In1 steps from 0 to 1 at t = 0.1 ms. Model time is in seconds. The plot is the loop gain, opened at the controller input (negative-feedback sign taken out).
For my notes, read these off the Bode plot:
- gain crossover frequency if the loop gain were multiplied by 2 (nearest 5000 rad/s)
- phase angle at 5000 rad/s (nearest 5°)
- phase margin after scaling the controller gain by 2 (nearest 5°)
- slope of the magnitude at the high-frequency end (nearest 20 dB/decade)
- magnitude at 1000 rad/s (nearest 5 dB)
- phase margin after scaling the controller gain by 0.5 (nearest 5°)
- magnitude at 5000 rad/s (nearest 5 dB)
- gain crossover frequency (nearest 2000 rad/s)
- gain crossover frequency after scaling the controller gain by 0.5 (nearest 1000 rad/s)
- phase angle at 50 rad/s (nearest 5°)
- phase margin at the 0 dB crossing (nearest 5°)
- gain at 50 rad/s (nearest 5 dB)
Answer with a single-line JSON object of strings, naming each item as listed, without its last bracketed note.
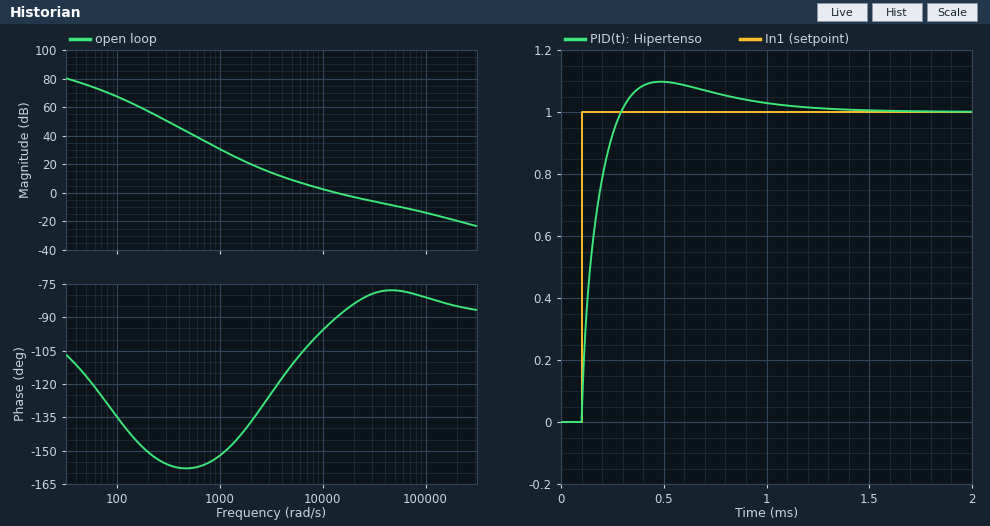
{"gain crossover frequency if the loop gain were multiplied by 2": "30000 rad/s", "phase angle at 5000 rad/s": "-110°", "phase margin after scaling the controller gain by 2": "100°", "slope of the magnitude at the high-frequency end": "-20 dB/decade", "magnitude at 1000 rad/s": "30 dB", "phase margin after scaling the controller gain by 0.5": "75°", "magnitude at 5000 rad/s": "10 dB", "gain crossover frequency": "14000 rad/s", "gain crossover frequency after scaling the controller gain by 0.5": "7000 rad/s", "phase angle at 50 rad/s": "-115°", "phase margin at the 0 dB crossing": "90°", "gain at 50 rad/s": "75 dB"}
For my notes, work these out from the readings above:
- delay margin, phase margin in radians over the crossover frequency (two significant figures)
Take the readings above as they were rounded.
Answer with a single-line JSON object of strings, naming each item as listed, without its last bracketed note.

{"delay margin, phase margin in radians over the crossover frequency": "0.00011 s"}
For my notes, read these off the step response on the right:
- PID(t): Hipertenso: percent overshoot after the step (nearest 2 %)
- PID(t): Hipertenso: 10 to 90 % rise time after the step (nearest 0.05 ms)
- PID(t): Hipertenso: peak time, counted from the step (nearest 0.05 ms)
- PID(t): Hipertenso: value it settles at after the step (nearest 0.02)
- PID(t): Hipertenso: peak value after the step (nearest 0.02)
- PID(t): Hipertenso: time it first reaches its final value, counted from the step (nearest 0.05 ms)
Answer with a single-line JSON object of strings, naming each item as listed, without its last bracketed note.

{"PID(t): Hipertenso: percent overshoot after the step": "10 %", "PID(t): Hipertenso: 10 to 90 % rise time after the step": "0.15 ms", "PID(t): Hipertenso: peak time, counted from the step": "0.40 ms", "PID(t): Hipertenso: value it settles at after the step": "1.00", "PID(t): Hipertenso: peak value after the step": "1.10", "PID(t): Hipertenso: time it first reaches its final value, counted from the step": "0.20 ms"}
